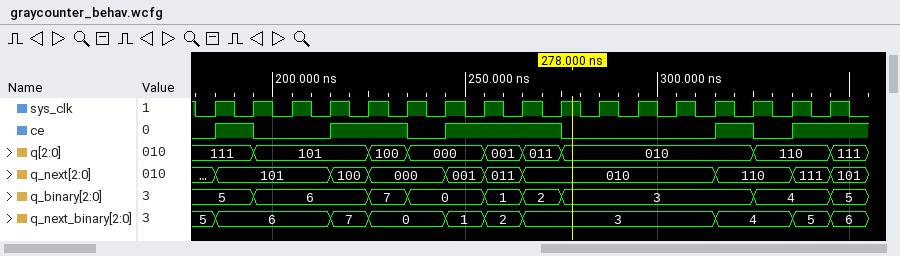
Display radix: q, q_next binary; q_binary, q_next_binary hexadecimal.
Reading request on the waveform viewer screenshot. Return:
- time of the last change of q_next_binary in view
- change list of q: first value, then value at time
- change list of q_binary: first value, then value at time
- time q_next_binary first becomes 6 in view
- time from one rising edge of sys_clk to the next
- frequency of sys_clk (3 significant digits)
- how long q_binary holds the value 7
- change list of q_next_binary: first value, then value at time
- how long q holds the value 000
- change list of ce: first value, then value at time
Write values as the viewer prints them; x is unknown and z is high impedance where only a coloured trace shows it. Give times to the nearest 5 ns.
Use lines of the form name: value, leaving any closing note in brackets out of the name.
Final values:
time of the last change of q_next_binary in view: 345 ns
change list of q: first value, then value at time: 111, 101 at 195 ns, 100 at 225 ns, 000 at 235 ns, 001 at 255 ns, 011 at 265 ns, 010 at 275 ns, 110 at 325 ns, 111 at 345 ns
change list of q_binary: first value, then value at time: 5, 6 at 195 ns, 7 at 225 ns, 0 at 235 ns, 1 at 255 ns, 2 at 265 ns, 3 at 275 ns, 4 at 325 ns, 5 at 345 ns
time q_next_binary first becomes 6 in view: 185 ns
time from one rising edge of sys_clk to the next: 10 ns
frequency of sys_clk: 100 MHz
how long q_binary holds the value 7: 10 ns
change list of q_next_binary: first value, then value at time: 5, 6 at 185 ns, 7 at 215 ns, 0 at 225 ns, 1 at 245 ns, 2 at 255 ns, 3 at 265 ns, 4 at 315 ns, 5 at 335 ns, 6 at 345 ns
how long q holds the value 000: 20 ns
change list of ce: first value, then value at time: 0, 1 at 185 ns, 0 at 195 ns, 1 at 215 ns, 0 at 235 ns, 1 at 245 ns, 0 at 275 ns, 1 at 315 ns, 0 at 325 ns, 1 at 335 ns
